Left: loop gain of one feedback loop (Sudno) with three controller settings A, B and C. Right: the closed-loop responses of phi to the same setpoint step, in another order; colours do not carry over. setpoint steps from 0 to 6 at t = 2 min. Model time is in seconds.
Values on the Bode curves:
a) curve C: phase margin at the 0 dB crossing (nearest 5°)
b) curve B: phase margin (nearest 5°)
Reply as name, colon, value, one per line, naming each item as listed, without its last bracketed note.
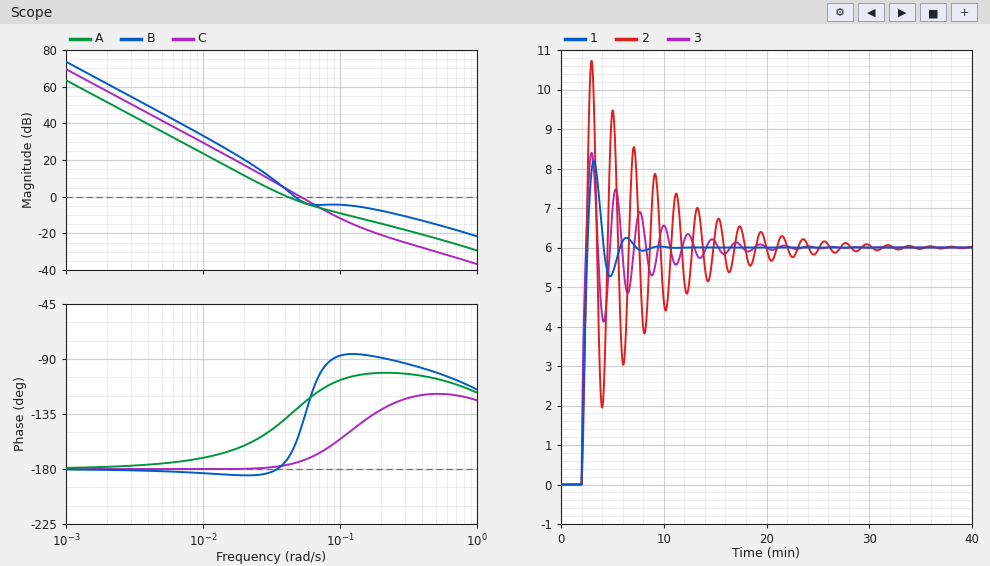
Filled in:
curve C: phase margin at the 0 dB crossing: 5°
curve B: phase margin: 20°
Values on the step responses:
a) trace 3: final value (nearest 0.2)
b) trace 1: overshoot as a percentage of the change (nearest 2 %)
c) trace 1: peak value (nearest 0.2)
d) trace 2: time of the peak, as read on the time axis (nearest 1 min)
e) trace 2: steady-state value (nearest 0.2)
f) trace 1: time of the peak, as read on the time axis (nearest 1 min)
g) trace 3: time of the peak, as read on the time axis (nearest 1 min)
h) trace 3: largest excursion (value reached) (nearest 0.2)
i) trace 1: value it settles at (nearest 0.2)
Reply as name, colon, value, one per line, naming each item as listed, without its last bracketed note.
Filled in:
trace 3: final value: 6.0
trace 1: overshoot as a percentage of the change: 36 %
trace 1: peak value: 8.2
trace 2: time of the peak, as read on the time axis: 3 min
trace 2: steady-state value: 6.0
trace 1: time of the peak, as read on the time axis: 3 min
trace 3: time of the peak, as read on the time axis: 3 min
trace 3: largest excursion (value reached): 8.4
trace 1: value it settles at: 6.0
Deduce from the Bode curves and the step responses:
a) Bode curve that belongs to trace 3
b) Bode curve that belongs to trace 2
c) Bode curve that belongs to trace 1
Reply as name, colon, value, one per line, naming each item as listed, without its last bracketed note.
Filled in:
Bode curve that belongs to trace 3: B
Bode curve that belongs to trace 2: C
Bode curve that belongs to trace 1: A
